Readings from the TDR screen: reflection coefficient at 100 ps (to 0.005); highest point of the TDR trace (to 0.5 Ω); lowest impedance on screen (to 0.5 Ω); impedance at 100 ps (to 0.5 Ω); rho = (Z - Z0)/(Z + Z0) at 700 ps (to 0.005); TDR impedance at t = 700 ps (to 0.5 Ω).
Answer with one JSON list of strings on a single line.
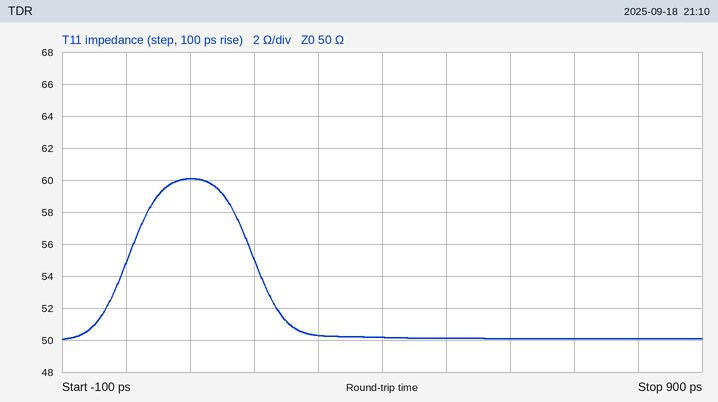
["+0.090", "60.0 Ω", "50.0 Ω", "60.0 Ω", "0.000", "50.0 Ω"]
